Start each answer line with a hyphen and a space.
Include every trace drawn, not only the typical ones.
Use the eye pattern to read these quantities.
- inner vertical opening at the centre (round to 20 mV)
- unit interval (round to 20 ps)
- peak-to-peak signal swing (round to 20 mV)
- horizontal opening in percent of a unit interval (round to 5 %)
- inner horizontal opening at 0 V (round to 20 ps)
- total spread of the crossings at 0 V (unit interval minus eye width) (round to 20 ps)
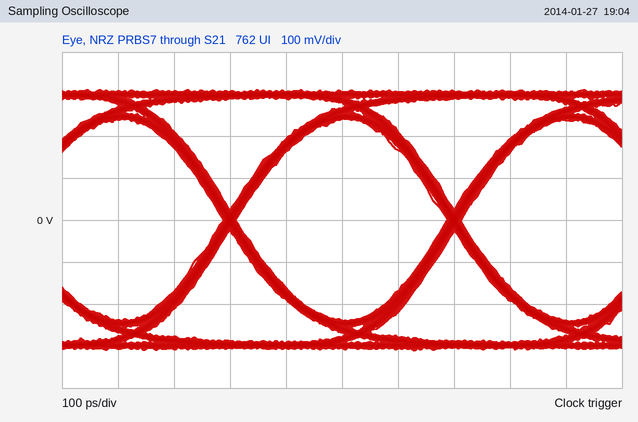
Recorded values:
- 480 mV
- 400 ps
- 620 mV
- 95 %
- 380 ps
- 20 ps
